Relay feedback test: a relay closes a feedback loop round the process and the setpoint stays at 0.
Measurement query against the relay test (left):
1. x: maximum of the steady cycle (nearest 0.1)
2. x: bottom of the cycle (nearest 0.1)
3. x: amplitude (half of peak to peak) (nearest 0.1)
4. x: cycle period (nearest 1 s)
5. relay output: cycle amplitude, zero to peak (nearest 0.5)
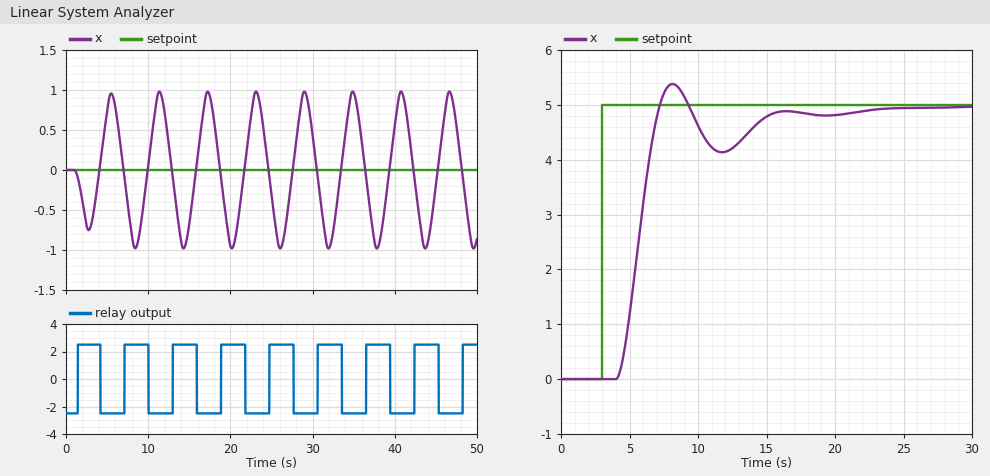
1.0
-1.0
1.0
6 s
2.5
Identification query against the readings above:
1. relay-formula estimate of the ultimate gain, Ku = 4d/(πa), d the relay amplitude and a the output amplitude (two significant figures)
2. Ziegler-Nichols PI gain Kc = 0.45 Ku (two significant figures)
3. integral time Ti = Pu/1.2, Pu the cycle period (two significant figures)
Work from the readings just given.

3.2
1.4
5.0 s
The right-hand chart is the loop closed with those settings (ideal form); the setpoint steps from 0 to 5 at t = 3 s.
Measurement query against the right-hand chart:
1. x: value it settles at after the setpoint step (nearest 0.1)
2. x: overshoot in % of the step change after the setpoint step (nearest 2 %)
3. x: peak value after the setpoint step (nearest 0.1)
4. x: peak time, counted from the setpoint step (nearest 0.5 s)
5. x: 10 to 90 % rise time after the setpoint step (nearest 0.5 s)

5.0
8 %
5.4
5.0 s
2.0 s
